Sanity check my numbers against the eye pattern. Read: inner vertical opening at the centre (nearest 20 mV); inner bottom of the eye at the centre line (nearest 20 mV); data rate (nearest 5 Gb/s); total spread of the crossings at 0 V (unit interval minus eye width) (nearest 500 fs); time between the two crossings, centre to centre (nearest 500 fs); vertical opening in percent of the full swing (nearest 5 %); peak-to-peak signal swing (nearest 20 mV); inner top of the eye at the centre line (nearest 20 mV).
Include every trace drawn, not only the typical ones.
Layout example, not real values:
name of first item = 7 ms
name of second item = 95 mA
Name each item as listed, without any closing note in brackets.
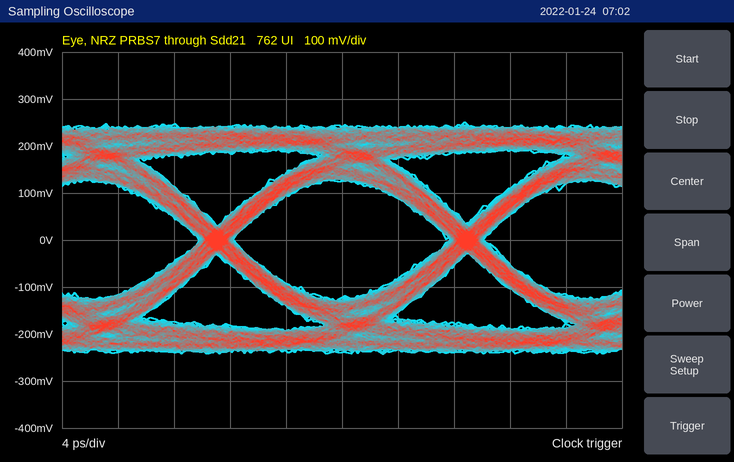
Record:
inner vertical opening at the centre = 240 mV
inner bottom of the eye at the centre line = -120 mV
data rate = 55 Gb/s
total spread of the crossings at 0 V (unit interval minus eye width) = 2.5 ps
time between the two crossings, centre to centre = 18.0 ps
vertical opening in percent of the full swing = 50 %
peak-to-peak signal swing = 500 mV
inner top of the eye at the centre line = 120 mV
